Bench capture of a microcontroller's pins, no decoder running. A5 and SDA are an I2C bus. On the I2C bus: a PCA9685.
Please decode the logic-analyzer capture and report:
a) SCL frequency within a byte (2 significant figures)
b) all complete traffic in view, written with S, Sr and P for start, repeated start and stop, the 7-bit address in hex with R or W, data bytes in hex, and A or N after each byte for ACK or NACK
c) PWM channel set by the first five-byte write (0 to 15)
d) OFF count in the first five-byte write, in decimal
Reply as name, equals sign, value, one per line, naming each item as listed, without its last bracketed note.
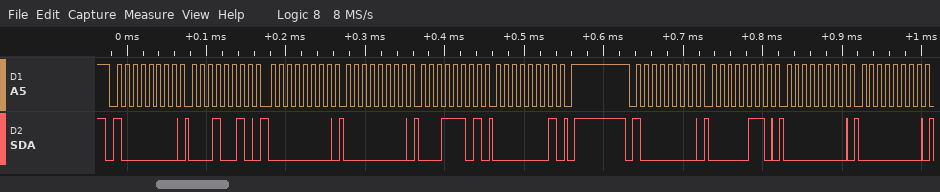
SCL frequency within a byte = 100 kHz
all complete traffic in view, written with S, Sr and P for start, repeated start and stop, the 7-bit address in hex with R or W, data bytes in hex, and A or N after each byte for ACK or NACK = S 40W A 12 A 00 A 00 A 1D A 01 A P S 40W A 06 A 00 A 00 A
PWM channel set by the first five-byte write = 3
OFF count in the first five-byte write, in decimal = 285
